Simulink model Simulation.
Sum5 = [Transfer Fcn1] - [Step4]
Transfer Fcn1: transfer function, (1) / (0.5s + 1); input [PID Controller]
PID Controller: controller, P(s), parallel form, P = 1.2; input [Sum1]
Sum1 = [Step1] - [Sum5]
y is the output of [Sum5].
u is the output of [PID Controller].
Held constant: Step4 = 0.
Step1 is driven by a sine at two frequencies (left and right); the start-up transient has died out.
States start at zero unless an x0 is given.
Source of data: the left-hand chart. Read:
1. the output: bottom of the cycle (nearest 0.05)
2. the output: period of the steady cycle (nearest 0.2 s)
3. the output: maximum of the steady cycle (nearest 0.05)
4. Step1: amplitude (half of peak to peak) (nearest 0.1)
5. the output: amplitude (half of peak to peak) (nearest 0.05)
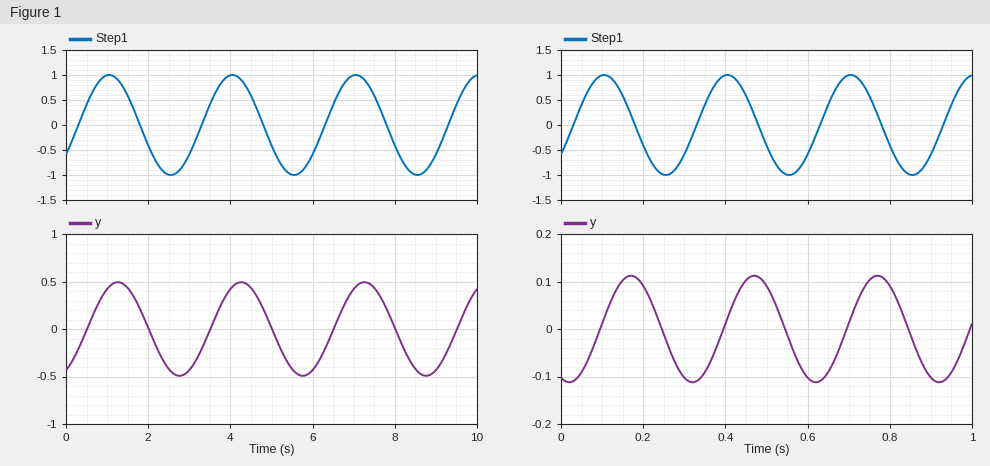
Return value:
-0.50
3.0 s
0.50
1.0
0.50
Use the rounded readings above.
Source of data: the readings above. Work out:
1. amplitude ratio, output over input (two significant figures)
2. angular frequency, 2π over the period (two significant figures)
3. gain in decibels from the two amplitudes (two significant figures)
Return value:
0.50
2.1 rad/s
-6.0 dB
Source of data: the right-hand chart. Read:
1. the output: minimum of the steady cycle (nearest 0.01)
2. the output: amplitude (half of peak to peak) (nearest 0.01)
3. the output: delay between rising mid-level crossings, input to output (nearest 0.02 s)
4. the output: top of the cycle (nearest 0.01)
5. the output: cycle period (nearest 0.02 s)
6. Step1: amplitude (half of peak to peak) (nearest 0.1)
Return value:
-0.11
0.11
0.06 s
0.11
0.30 s
1.0
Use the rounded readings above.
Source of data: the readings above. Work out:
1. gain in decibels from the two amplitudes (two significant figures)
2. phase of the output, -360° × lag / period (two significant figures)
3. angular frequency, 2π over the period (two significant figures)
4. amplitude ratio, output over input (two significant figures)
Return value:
-19 dB
-72°
21 rad/s
0.11
